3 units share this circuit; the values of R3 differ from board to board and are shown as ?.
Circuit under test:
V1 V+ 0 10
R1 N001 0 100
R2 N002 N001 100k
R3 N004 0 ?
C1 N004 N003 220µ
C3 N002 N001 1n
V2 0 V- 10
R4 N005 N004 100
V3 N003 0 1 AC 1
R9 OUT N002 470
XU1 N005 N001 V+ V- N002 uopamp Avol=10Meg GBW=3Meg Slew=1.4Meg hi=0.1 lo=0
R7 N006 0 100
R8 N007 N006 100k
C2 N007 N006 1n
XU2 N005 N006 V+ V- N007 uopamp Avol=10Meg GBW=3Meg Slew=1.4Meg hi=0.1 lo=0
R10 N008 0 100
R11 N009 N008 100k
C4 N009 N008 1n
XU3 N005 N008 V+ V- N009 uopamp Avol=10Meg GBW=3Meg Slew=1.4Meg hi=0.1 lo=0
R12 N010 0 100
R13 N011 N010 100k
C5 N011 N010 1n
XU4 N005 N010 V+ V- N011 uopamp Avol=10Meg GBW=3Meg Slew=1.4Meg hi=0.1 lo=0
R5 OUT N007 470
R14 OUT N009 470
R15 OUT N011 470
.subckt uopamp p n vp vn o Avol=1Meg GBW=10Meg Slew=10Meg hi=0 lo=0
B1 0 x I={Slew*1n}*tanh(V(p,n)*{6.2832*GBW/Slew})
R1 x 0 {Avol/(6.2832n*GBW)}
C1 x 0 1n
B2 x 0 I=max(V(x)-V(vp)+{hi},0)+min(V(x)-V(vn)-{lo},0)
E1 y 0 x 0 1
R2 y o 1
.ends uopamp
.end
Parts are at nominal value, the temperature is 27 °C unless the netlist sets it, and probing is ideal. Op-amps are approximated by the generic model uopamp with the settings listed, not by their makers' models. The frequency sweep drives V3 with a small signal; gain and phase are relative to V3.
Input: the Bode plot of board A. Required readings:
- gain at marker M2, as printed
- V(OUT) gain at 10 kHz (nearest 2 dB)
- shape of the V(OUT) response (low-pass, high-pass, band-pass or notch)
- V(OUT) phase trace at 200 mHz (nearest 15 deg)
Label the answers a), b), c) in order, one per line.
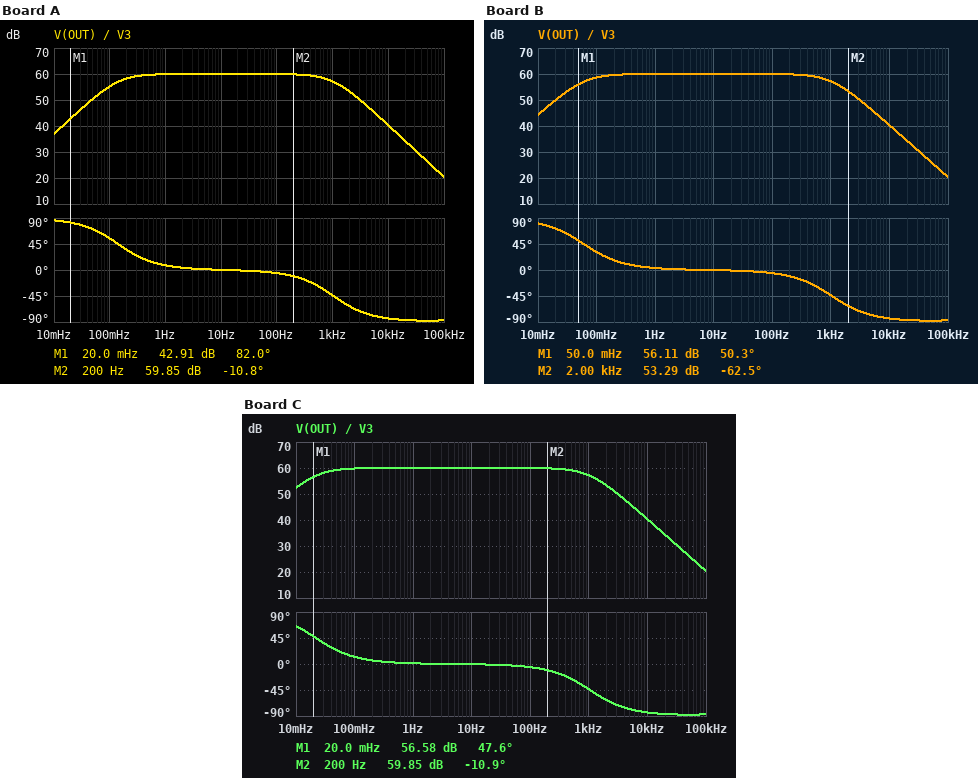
a) 59.85 dB
b) 40 dB
c) band-pass
d) 30 deg
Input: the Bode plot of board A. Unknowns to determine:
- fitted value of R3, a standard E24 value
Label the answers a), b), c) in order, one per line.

a) 5.1 kΩ
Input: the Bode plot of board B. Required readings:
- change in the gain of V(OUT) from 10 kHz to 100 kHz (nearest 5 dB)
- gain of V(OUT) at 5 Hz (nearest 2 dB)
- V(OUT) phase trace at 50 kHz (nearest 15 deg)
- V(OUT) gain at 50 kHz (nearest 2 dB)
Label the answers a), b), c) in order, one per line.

a) -20 dB
b) 60 dB
c) -90 deg
d) 26 dB
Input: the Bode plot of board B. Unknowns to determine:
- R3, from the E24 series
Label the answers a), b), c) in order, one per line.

a) 12 kΩ
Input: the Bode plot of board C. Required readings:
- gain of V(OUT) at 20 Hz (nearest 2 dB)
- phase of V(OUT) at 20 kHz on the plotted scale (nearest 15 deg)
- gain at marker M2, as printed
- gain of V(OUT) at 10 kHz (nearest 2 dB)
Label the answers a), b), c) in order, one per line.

a) 60 dB
b) -90 deg
c) 59.85 dB
d) 40 dB
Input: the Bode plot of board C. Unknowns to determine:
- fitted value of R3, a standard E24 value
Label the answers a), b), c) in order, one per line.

a) 33 kΩ
